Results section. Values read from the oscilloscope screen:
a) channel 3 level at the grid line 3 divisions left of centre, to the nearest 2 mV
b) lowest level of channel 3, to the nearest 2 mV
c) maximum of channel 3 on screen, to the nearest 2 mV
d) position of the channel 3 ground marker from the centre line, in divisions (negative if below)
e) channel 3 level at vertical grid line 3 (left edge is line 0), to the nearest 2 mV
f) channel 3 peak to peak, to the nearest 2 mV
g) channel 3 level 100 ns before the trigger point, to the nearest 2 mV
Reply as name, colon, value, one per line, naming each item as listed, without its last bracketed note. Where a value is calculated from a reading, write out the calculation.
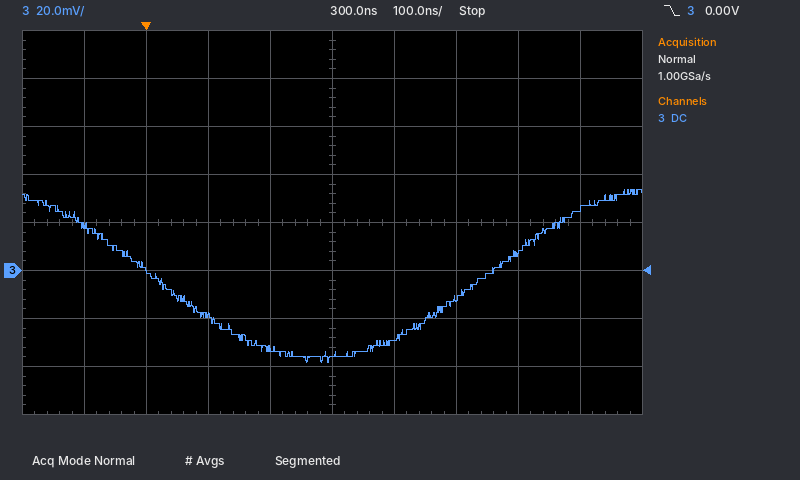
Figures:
channel 3 level at the grid line 3 divisions left of centre, to the nearest 2 mV: 0 mV
lowest level of channel 3, to the nearest 2 mV: -38 mV
maximum of channel 3 on screen, to the nearest 2 mV: 34 mV
position of the channel 3 ground marker from the centre line, in divisions: -1.0 div
channel 3 level at vertical grid line 3 (left edge is line 0), to the nearest 2 mV: -18 mV
channel 3 peak to peak, to the nearest 2 mV: 34 mV − (-38 mV) = 72 mV
channel 3 level 100 ns before the trigger point, to the nearest 2 mV: 18 mV
